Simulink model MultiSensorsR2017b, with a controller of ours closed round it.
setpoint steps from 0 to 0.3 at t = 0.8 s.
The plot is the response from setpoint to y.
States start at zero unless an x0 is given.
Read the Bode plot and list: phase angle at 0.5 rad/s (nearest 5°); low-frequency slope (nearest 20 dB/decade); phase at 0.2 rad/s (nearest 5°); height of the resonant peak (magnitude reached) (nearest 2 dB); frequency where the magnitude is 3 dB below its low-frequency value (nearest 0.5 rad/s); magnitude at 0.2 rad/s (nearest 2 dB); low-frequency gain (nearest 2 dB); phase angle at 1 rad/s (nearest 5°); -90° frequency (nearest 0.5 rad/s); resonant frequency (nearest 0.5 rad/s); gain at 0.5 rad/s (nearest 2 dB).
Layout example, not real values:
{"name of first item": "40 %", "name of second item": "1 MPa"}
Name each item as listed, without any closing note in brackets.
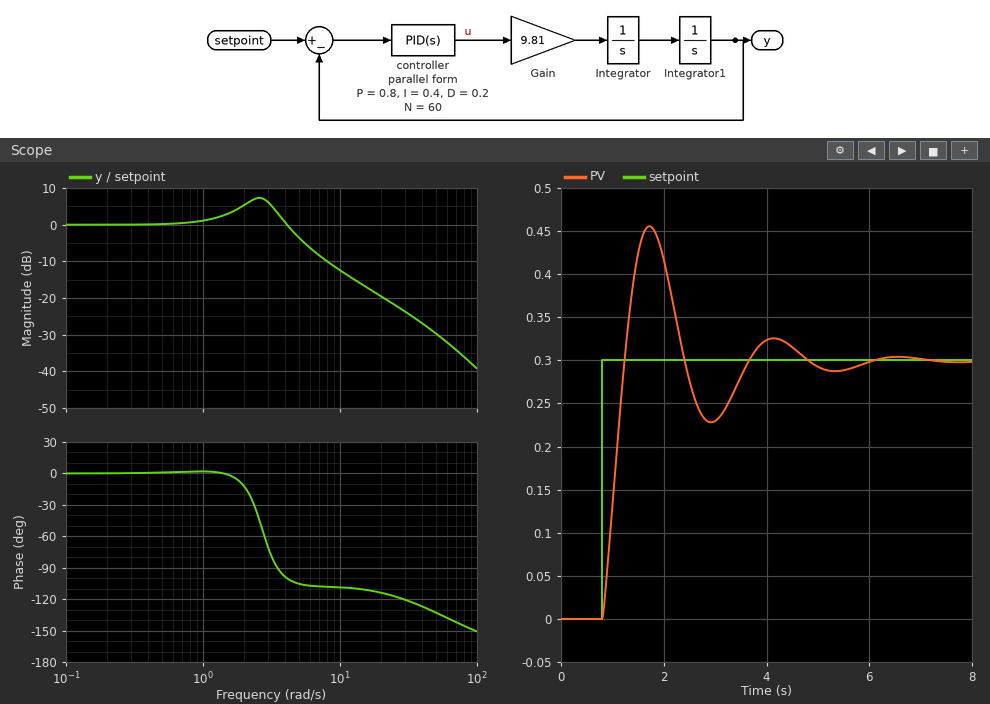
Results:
{"phase angle at 0.5 rad/s": "0°", "low-frequency slope": "0 dB/decade", "phase at 0.2 rad/s": "0°", "height of the resonant peak (magnitude reached)": "8 dB", "frequency where the magnitude is 3 dB below its low-frequency value": "5.0 rad/s", "magnitude at 0.2 rad/s": "0 dB", "low-frequency gain": "0 dB", "phase angle at 1 rad/s": "0°", "-90° frequency": "3.5 rad/s", "resonant frequency": "2.5 rad/s", "gain at 0.5 rad/s": "0 dB"}
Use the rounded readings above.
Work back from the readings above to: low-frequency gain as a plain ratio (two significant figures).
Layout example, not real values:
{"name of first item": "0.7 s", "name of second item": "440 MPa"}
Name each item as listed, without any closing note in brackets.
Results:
{"low-frequency gain as a plain ratio": "1.0"}
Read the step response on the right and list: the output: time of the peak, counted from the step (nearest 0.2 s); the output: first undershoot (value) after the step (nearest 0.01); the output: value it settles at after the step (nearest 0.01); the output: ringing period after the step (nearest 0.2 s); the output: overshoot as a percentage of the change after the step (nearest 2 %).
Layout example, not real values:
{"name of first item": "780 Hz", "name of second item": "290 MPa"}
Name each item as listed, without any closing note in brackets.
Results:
{"the output: time of the peak, counted from the step": "1.0 s", "the output: first undershoot (value) after the step": "0.23", "the output: value it settles at after the step": "0.30", "the output: ringing period after the step": "2.4 s", "the output: overshoot as a percentage of the change after the step": "52 %"}
